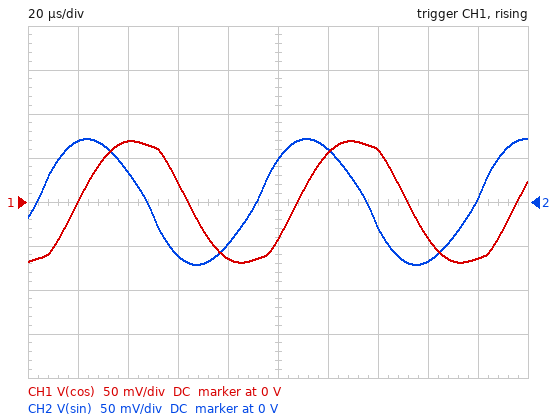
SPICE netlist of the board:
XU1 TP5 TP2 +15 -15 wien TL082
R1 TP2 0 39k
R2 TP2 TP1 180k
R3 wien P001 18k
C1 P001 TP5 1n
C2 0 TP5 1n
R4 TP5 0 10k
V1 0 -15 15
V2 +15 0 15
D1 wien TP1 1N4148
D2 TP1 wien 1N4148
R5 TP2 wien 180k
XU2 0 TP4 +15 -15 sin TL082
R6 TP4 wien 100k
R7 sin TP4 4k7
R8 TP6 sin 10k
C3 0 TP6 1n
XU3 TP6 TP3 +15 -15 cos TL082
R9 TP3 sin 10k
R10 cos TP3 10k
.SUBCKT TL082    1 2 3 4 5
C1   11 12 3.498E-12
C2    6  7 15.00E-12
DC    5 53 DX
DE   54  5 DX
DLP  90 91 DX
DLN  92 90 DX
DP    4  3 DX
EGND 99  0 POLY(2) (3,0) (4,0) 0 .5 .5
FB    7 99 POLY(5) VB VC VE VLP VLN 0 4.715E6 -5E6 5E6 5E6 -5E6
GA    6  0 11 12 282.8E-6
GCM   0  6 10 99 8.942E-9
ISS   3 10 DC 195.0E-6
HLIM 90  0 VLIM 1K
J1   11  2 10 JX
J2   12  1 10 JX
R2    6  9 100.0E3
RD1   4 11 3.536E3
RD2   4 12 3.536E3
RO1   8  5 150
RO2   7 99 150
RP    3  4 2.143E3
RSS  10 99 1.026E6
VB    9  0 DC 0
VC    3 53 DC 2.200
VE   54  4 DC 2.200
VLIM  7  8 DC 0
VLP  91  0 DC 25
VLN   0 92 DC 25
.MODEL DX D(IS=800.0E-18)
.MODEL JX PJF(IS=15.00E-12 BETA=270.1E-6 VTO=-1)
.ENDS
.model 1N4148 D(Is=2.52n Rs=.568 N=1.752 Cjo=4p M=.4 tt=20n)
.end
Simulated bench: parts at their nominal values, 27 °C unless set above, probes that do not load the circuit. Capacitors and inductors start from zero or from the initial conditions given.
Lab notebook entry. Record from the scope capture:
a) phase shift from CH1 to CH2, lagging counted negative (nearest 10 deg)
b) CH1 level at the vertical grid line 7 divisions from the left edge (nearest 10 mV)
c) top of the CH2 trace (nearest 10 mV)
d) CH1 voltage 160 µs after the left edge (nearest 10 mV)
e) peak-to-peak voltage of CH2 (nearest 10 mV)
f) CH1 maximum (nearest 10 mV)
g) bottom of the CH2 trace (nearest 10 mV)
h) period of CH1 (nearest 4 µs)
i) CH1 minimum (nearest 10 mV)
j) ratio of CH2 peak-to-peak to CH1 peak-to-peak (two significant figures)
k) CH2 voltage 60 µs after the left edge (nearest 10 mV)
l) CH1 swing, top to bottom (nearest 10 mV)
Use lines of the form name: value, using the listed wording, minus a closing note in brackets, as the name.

phase shift from CH1 to CH2, lagging counted negative: 70 deg
CH1 level at the vertical grid line 7 divisions from the left edge: 60 mV
top of the CH2 trace: 70 mV
CH1 voltage 160 µs after the left edge: -40 mV
peak-to-peak voltage of CH2: 140 mV
CH1 maximum: 70 mV
bottom of the CH2 trace: -70 mV
period of CH1: 88 µs
CH1 minimum: -70 mV
ratio of CH2 peak-to-peak to CH1 peak-to-peak: 1.0
CH2 voltage 60 µs after the left edge: -60 mV
CH1 swing, top to bottom: 140 mV
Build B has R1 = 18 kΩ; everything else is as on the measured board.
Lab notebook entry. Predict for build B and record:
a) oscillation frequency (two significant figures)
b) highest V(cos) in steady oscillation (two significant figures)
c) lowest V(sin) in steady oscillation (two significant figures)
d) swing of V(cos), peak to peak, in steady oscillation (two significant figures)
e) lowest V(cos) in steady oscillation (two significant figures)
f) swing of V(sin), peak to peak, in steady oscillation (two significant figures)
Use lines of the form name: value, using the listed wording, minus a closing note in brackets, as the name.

oscillation frequency: 9.2 kHz
highest V(cos) in steady oscillation: 980 mV
lowest V(sin) in steady oscillation: -630 mV
swing of V(cos), peak to peak, in steady oscillation: 2.0 V
lowest V(cos) in steady oscillation: -980 mV
swing of V(sin), peak to peak, in steady oscillation: 1.3 V
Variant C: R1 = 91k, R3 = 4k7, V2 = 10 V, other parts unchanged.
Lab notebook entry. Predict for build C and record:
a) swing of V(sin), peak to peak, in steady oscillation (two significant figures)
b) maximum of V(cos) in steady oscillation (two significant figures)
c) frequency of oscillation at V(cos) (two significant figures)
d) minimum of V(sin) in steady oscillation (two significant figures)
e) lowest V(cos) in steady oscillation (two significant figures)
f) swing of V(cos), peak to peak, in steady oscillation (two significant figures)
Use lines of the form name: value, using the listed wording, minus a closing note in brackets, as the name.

swing of V(sin), peak to peak, in steady oscillation: 70 mV
maximum of V(cos) in steady oscillation: 34 mV
frequency of oscillation at V(cos): 21 kHz
minimum of V(sin) in steady oscillation: -35 mV
lowest V(cos) in steady oscillation: -34 mV
swing of V(cos), peak to peak, in steady oscillation: 68 mV
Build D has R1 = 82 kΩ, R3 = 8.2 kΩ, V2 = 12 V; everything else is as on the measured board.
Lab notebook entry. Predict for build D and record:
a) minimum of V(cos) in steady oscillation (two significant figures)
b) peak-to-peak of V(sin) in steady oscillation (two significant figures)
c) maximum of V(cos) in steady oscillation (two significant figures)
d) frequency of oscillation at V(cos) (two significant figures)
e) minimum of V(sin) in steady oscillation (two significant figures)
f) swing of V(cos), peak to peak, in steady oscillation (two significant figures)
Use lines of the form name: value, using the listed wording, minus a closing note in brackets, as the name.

minimum of V(cos) in steady oscillation: -21 mV
peak-to-peak of V(sin) in steady oscillation: 44 mV
maximum of V(cos) in steady oscillation: 21 mV
frequency of oscillation at V(cos): 16 kHz
minimum of V(sin) in steady oscillation: -22 mV
swing of V(cos), peak to peak, in steady oscillation: 42 mV
